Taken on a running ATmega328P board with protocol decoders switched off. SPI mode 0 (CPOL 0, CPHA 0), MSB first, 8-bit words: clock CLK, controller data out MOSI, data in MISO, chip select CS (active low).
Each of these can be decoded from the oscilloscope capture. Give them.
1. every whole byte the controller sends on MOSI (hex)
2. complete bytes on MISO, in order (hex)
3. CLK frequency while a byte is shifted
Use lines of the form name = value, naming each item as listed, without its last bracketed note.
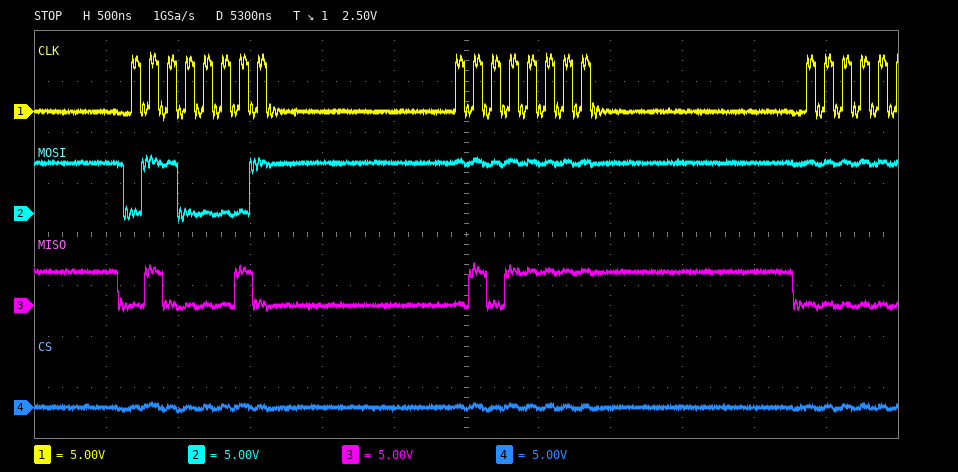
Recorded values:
every whole byte the controller sends on MOSI = 61 FF
complete bytes on MISO, in order = 42 5F
CLK frequency while a byte is shifted = 8 MHz
